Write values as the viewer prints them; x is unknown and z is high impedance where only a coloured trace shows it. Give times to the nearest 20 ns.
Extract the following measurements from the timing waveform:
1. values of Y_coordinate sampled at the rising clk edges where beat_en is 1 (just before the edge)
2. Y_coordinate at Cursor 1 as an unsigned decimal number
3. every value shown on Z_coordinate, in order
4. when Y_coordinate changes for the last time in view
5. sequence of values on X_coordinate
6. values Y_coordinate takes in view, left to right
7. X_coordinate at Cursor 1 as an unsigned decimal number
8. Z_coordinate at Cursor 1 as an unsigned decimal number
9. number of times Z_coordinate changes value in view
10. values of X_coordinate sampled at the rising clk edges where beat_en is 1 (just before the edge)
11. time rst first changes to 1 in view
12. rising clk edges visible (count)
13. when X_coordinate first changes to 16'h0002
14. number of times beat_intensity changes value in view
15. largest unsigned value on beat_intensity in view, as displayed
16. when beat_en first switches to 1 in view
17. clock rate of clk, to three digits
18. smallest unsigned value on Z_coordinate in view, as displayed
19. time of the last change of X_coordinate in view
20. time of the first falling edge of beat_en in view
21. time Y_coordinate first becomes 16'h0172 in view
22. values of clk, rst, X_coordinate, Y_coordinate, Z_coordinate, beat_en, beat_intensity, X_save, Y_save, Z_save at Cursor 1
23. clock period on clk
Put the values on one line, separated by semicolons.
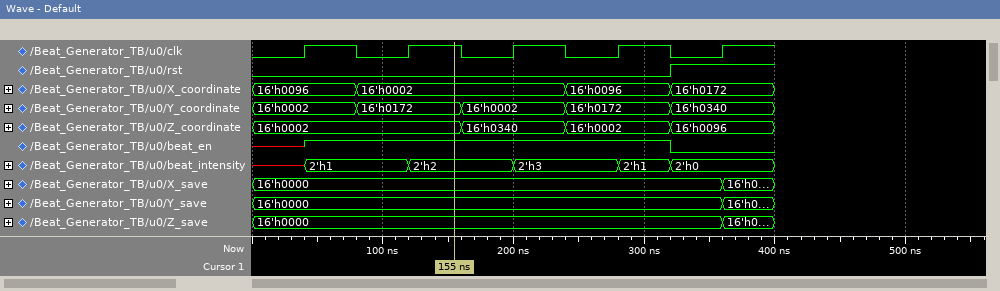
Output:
16'h0172, 16'h0002, 16'h0172; 370; 16'h0002, 16'h0340, 16'h0002, 16'h0096; 320 ns; 16'h0096, 16'h0002, 16'h0096, 16'h0172; 16'h0002, 16'h0172, 16'h0002, 16'h0172, 16'h0340; 2; 2; 3; 16'h0002, 16'h0002, 16'h0096; 320 ns; 5; 80 ns; 5; 2'h3; 40 ns; 12.5 MHz; 16'h0002; 320 ns; 320 ns; 80 ns; clk=1, rst=0, X_coordinate=16'h0002, Y_coordinate=16'h0172, Z_coordinate=16'h0002, beat_en=1, beat_intensity=2'h2, X_save=16'h0000, Y_save=16'h0000, Z_save=16'h0000; 80 ns
